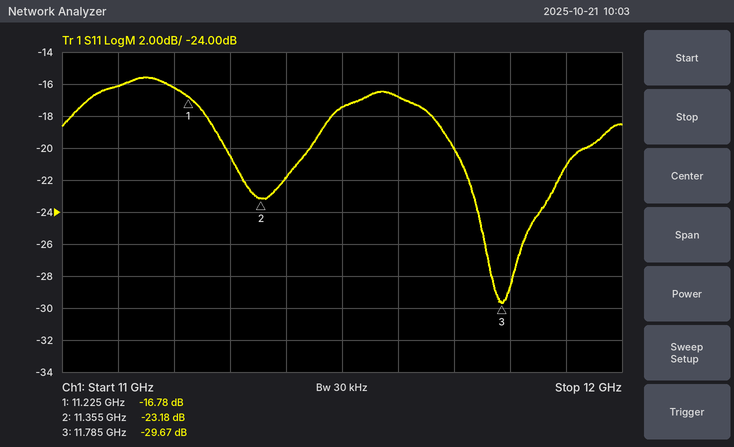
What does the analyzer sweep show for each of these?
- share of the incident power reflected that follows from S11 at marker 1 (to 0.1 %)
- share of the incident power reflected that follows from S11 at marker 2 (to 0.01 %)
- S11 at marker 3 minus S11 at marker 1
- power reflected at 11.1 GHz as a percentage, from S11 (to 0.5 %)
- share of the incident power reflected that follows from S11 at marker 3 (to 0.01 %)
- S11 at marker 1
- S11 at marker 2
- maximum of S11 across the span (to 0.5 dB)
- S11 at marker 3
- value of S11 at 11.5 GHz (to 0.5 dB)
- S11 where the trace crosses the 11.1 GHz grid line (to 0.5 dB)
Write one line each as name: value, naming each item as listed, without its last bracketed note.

share of the incident power reflected that follows from S11 at marker 1: 2.1 %
share of the incident power reflected that follows from S11 at marker 2: 0.48 %
S11 at marker 3 minus S11 at marker 1: -12.89 dB
power reflected at 11.1 GHz as a percentage, from S11: 2.5 %
share of the incident power reflected that follows from S11 at marker 3: 0.11 %
S11 at marker 1: -16.78 dB
S11 at marker 2: -23.18 dB
maximum of S11 across the span: -15.5 dB
S11 at marker 3: -29.67 dB
value of S11 at 11.5 GHz: -17.5 dB
S11 where the trace crosses the 11.1 GHz grid line: -16.0 dB
